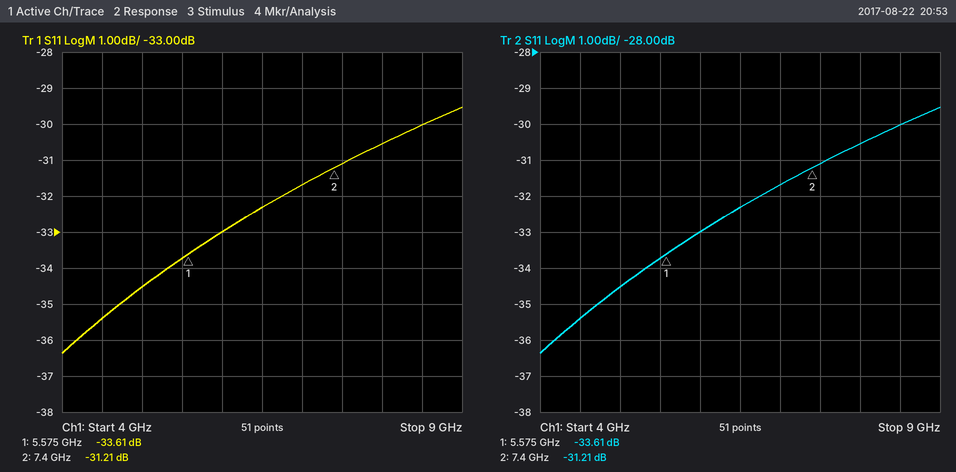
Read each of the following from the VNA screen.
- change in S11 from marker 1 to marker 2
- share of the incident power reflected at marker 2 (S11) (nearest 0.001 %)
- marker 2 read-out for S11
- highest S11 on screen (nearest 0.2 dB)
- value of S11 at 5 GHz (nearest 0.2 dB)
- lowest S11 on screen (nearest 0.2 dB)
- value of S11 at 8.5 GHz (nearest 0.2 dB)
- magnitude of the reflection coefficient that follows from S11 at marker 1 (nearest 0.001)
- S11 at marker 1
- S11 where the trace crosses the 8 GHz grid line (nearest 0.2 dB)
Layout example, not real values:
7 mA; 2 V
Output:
2.40 dB; 0.076 %; -31.21 dB; -29.6 dB; -34.6 dB; -36.4 dB; -30.0 dB; 0.021; -33.61 dB; -30.6 dB
